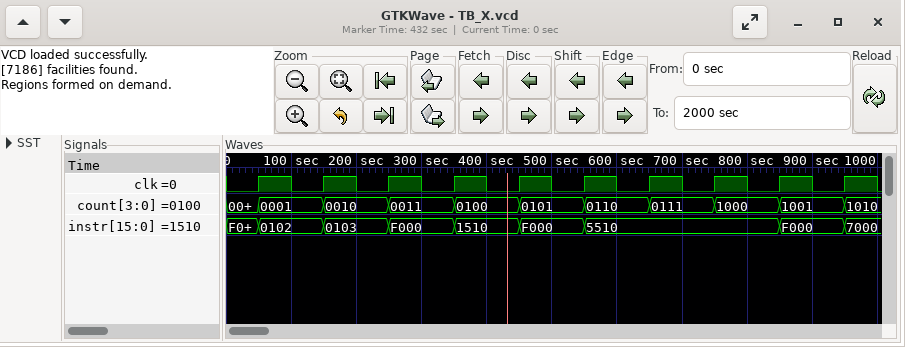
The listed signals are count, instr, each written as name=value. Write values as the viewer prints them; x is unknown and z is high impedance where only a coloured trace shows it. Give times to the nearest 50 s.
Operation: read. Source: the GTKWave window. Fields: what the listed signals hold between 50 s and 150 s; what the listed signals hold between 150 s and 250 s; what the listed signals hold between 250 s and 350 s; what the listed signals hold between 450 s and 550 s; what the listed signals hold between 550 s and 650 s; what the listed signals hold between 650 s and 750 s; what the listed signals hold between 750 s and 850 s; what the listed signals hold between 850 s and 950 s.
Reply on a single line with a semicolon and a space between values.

count=0001, instr=0102; count=0010, instr=0103; count=0011, instr=F000; count=0101, instr=F000; count=0110, instr=5510; count=0111, instr=5510; count=1000, instr=5510; count=1001, instr=F000
